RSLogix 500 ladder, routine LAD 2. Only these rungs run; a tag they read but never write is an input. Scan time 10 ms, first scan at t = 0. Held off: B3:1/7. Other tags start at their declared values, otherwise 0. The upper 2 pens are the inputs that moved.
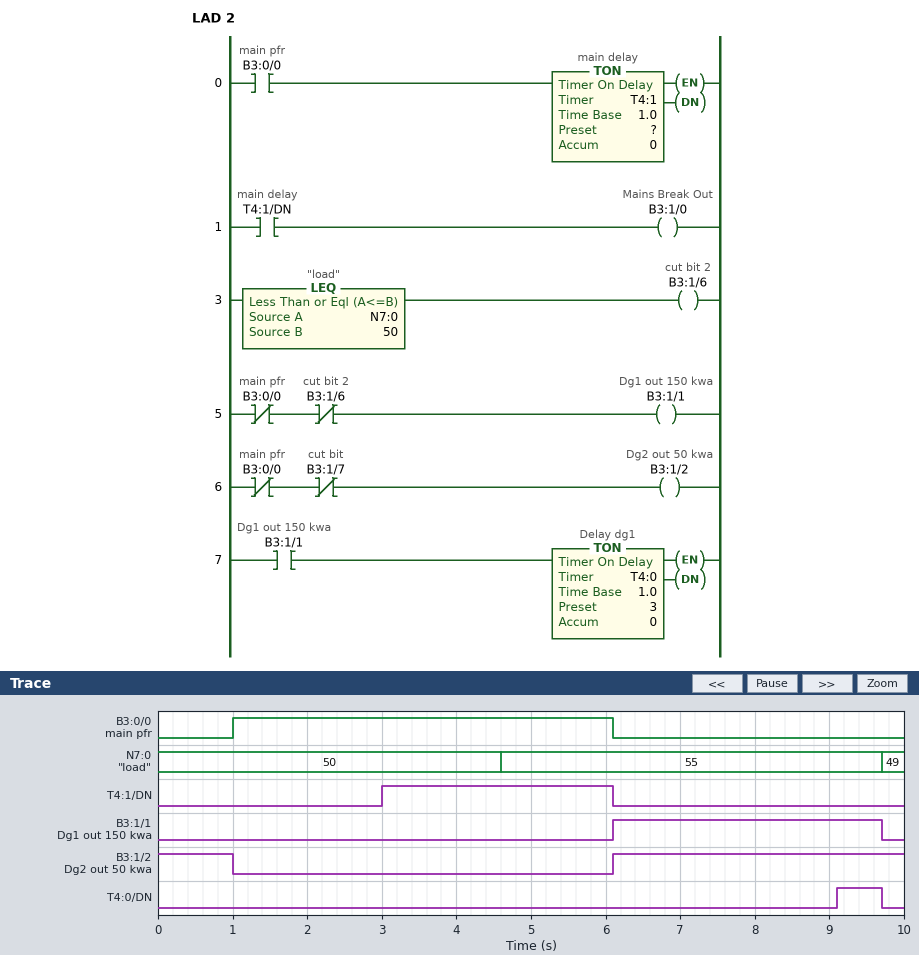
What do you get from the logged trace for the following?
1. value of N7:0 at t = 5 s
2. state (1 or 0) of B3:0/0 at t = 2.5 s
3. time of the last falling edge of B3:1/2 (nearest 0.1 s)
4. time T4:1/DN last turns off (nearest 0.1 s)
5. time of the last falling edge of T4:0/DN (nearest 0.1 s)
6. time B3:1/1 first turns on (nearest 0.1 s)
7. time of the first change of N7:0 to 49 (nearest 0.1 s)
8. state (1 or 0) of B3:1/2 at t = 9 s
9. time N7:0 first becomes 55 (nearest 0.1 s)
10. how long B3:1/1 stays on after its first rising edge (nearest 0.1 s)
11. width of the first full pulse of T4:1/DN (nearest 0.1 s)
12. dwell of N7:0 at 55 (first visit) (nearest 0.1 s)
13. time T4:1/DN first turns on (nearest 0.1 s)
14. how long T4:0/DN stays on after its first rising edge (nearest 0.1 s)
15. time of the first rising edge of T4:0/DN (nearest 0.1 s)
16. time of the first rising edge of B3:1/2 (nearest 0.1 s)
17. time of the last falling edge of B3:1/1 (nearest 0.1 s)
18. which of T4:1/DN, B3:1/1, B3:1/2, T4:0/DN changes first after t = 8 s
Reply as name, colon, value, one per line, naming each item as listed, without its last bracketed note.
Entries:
value of N7:0 at t = 5 s: 55
state (1 or 0) of B3:0/0 at t = 2.5 s: 1
time of the last falling edge of B3:1/2: 1.0 s
time T4:1/DN last turns off: 6.1 s
time of the last falling edge of T4:0/DN: 9.7 s
time B3:1/1 first turns on: 6.1 s
time of the first change of N7:0 to 49: 9.7 s
state (1 or 0) of B3:1/2 at t = 9 s: 1
time N7:0 first becomes 55: 4.6 s
how long B3:1/1 stays on after its first rising edge: 3.6 s
width of the first full pulse of T4:1/DN: 3.1 s
dwell of N7:0 at 55 (first visit): 5.1 s
time T4:1/DN first turns on: 3.0 s
how long T4:0/DN stays on after its first rising edge: 0.6 s
time of the first rising edge of T4:0/DN: 9.1 s
time of the first rising edge of B3:1/2: 6.1 s
time of the last falling edge of B3:1/1: 9.7 s
which of T4:1/DN, B3:1/1, B3:1/2, T4:0/DN changes first after t = 8 s: T4:0/DN
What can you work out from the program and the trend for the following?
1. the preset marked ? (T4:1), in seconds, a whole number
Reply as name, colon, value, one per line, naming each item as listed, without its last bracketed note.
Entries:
the preset marked ? (T4:1), in seconds, a whole number: 2 s
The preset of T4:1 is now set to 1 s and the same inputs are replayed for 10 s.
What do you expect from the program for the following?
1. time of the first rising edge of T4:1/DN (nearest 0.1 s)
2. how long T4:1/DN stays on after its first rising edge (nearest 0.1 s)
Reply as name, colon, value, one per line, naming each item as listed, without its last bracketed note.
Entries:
time of the first rising edge of T4:1/DN: 2.0 s
how long T4:1/DN stays on after its first rising edge: 4.1 s
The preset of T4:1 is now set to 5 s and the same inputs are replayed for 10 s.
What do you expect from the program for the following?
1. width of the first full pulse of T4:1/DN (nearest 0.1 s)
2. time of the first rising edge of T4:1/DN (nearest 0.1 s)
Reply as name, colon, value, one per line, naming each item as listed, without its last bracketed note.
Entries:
width of the first full pulse of T4:1/DN: 0.1 s
time of the first rising edge of T4:1/DN: 6.0 s
